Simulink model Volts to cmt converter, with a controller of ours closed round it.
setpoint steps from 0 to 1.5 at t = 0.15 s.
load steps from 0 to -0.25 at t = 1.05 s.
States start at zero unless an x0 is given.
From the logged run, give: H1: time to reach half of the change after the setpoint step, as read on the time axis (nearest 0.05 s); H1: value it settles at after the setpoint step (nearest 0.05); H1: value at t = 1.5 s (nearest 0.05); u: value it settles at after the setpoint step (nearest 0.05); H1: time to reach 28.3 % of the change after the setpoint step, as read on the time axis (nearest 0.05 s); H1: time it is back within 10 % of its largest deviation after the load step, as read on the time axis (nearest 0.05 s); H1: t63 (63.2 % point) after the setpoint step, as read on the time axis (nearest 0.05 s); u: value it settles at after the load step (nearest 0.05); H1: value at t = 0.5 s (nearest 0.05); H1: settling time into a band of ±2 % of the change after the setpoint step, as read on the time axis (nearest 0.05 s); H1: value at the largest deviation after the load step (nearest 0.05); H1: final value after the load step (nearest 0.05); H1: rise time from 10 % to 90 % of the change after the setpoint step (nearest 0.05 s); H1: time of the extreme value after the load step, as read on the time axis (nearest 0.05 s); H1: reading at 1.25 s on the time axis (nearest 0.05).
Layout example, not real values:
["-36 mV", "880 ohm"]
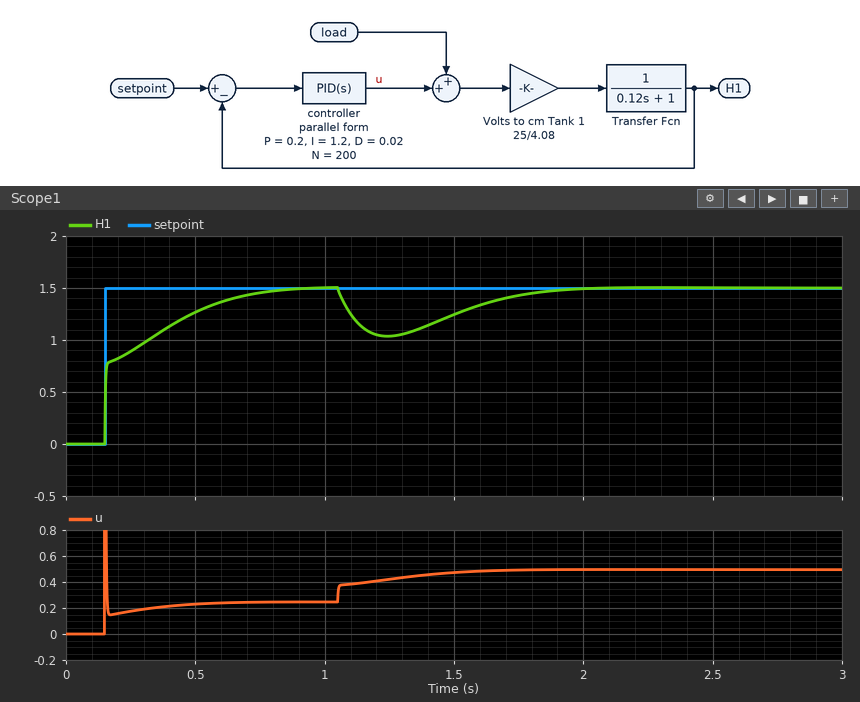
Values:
["0.15 s", "1.50", "1.25", "0.25", "0.15 s", "1.80 s", "0.30 s", "0.50", "1.25", "0.80 s", "1.05", "1.50", "0.45 s", "1.25 s", "1.05"]
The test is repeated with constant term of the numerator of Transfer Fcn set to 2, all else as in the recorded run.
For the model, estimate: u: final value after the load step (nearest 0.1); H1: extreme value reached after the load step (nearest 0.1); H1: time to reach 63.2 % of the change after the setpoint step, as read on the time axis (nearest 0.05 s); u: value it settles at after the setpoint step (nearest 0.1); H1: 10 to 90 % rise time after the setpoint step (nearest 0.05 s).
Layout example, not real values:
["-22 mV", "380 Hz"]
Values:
["0.4", "0.9", "0.15 s", "0.1", "0.30 s"]
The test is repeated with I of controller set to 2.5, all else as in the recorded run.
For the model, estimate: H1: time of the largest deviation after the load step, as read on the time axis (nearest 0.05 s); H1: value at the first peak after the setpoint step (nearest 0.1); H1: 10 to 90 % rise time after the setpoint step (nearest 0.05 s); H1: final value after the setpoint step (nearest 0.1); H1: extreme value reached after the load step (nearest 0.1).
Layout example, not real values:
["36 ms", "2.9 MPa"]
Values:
["1.20 s", "1.6", "0.25 s", "1.5", "1.1"]
